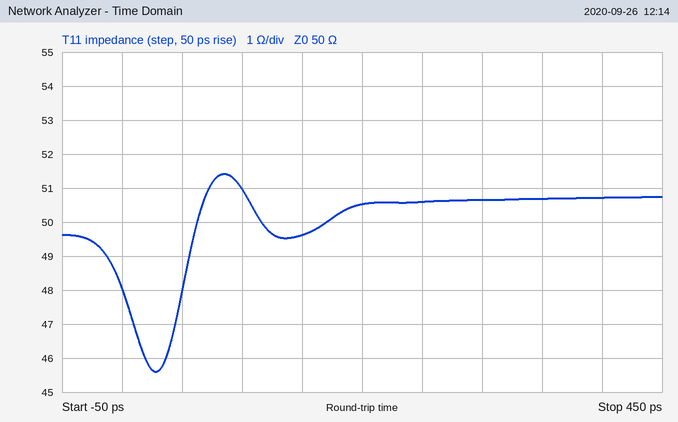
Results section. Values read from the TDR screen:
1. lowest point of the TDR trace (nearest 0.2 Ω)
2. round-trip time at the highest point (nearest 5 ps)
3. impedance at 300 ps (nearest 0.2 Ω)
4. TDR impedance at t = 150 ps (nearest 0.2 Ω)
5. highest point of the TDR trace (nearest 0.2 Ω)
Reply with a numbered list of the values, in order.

1. 45.6 Ω
2. 85 ps
3. 50.6 Ω
4. 49.6 Ω
5. 51.4 Ω
